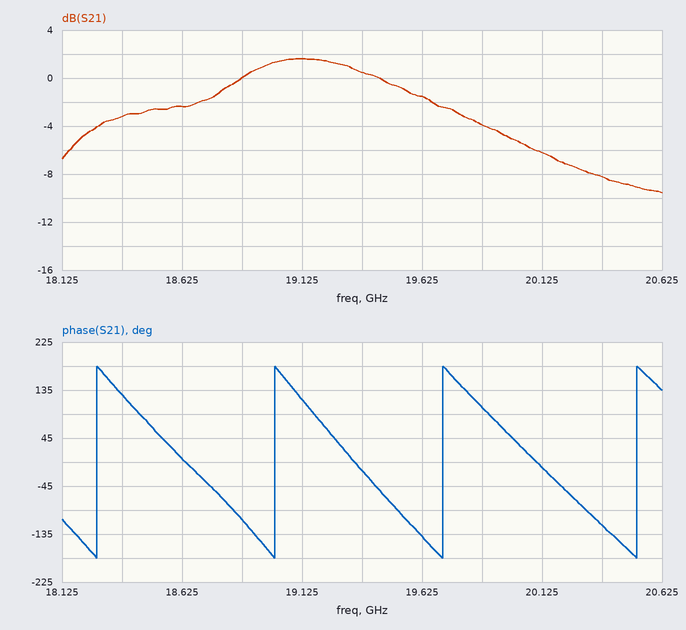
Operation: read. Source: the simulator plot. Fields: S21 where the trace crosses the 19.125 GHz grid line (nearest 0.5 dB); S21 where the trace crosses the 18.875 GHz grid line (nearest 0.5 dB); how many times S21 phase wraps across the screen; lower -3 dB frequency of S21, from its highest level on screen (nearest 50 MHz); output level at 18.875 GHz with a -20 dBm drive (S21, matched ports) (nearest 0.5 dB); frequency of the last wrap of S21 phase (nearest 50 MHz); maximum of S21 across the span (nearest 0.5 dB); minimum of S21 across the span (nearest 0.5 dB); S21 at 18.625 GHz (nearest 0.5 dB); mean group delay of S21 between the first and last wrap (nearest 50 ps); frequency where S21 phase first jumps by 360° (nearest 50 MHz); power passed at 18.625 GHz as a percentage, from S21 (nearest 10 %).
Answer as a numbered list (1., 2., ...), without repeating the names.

1. 1.5 dB
2. 0.0 dB
3. 4
4. 18.75 GHz
5. -20.0 dBm
6. 20.50 GHz
7. 1.5 dB
8. -9.5 dB
9. -2.5 dB
10. 1.35 ns
11. 18.25 GHz
12. 60 %
